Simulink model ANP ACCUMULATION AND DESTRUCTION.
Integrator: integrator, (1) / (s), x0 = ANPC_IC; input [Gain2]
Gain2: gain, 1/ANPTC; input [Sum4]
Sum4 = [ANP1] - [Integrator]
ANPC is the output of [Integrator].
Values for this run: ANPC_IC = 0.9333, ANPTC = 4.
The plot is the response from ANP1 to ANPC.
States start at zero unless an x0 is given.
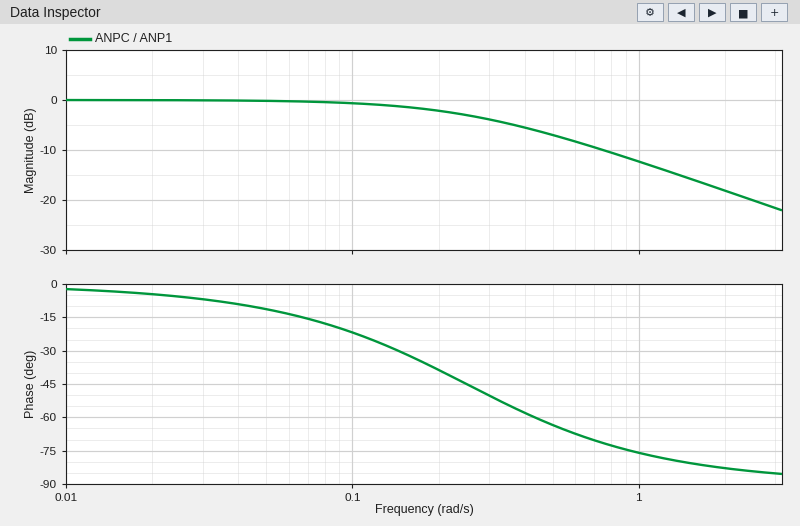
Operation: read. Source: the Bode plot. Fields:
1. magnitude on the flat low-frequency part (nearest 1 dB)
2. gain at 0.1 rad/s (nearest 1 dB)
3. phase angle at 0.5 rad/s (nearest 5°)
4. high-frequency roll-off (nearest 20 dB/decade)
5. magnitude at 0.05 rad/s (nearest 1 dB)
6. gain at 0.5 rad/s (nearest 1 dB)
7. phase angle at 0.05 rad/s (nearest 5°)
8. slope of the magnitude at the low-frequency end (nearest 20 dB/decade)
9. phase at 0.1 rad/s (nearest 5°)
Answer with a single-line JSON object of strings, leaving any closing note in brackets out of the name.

{"magnitude on the flat low-frequency part": "0 dB", "gain at 0.1 rad/s": "-1 dB", "phase angle at 0.5 rad/s": "-65°", "high-frequency roll-off": "-20 dB/decade", "magnitude at 0.05 rad/s": "0 dB", "gain at 0.5 rad/s": "-7 dB", "phase angle at 0.05 rad/s": "-10°", "slope of the magnitude at the low-frequency end": "0 dB/decade", "phase at 0.1 rad/s": "-20°"}
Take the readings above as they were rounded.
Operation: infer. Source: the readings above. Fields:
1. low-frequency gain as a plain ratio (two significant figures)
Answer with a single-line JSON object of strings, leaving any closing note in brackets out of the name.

{"low-frequency gain as a plain ratio": "1.0"}
